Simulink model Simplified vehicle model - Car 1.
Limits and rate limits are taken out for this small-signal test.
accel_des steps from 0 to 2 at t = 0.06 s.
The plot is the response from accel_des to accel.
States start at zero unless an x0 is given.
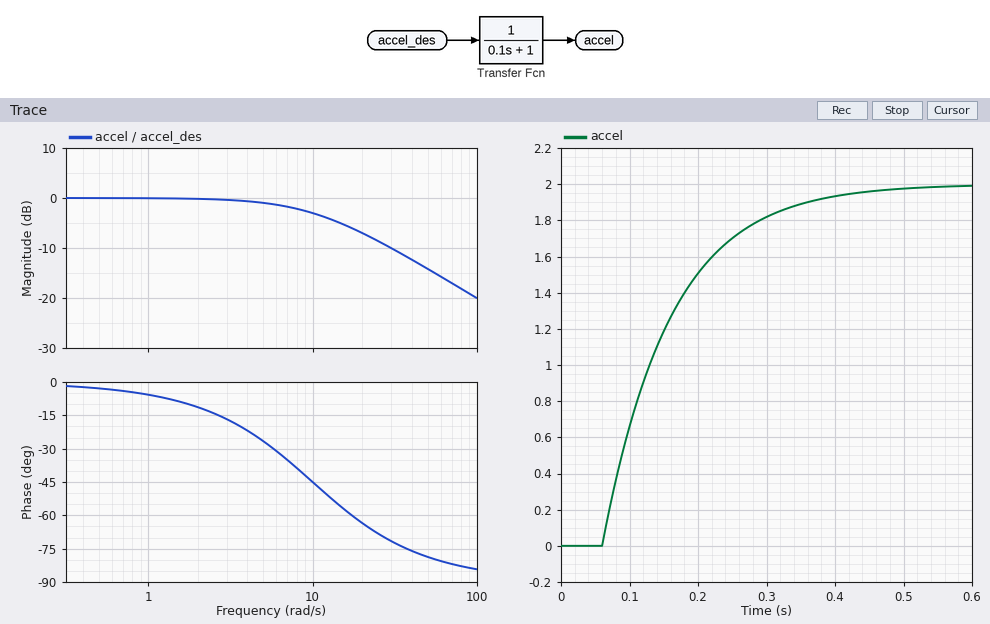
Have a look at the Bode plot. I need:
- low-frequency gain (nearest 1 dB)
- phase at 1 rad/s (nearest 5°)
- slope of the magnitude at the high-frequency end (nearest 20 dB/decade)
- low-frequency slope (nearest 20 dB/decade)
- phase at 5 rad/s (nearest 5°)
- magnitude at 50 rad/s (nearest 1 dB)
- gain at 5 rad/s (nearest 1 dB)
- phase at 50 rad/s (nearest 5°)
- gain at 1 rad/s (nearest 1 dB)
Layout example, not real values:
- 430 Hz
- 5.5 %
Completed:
- 0 dB
- -5°
- -20 dB/decade
- 0 dB/decade
- -25°
- -14 dB
- -1 dB
- -80°
- 0 dB
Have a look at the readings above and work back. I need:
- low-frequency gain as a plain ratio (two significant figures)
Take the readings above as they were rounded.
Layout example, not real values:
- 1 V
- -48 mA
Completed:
- 1.0
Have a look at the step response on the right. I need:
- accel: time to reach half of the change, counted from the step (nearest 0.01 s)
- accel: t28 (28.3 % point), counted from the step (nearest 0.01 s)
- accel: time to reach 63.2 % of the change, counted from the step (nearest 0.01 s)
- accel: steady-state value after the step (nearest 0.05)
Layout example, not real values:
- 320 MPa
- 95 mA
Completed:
- 0.07 s
- 0.03 s
- 0.10 s
- 2.00
